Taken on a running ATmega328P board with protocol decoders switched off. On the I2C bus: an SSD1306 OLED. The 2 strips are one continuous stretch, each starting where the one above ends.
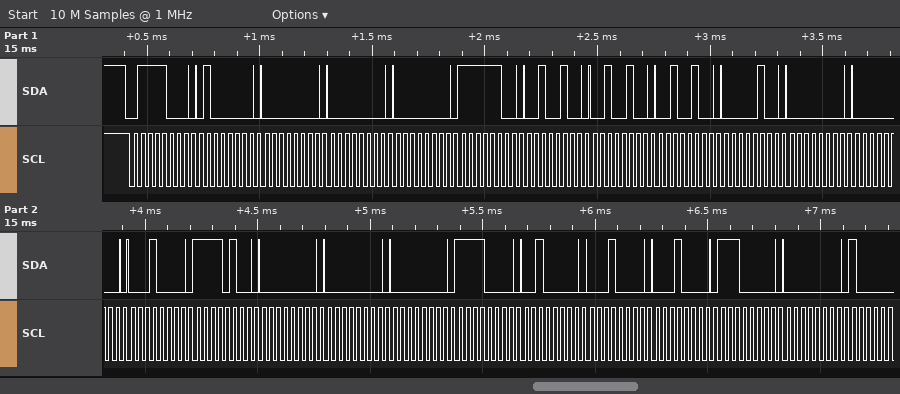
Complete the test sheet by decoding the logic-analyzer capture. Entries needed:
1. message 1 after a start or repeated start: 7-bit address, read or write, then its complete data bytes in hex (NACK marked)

0x3C write: 40 00 00 00 FC 24 24 24 04 00 00 10 F4 00 00 00 F0 20 10 10 E0 00
